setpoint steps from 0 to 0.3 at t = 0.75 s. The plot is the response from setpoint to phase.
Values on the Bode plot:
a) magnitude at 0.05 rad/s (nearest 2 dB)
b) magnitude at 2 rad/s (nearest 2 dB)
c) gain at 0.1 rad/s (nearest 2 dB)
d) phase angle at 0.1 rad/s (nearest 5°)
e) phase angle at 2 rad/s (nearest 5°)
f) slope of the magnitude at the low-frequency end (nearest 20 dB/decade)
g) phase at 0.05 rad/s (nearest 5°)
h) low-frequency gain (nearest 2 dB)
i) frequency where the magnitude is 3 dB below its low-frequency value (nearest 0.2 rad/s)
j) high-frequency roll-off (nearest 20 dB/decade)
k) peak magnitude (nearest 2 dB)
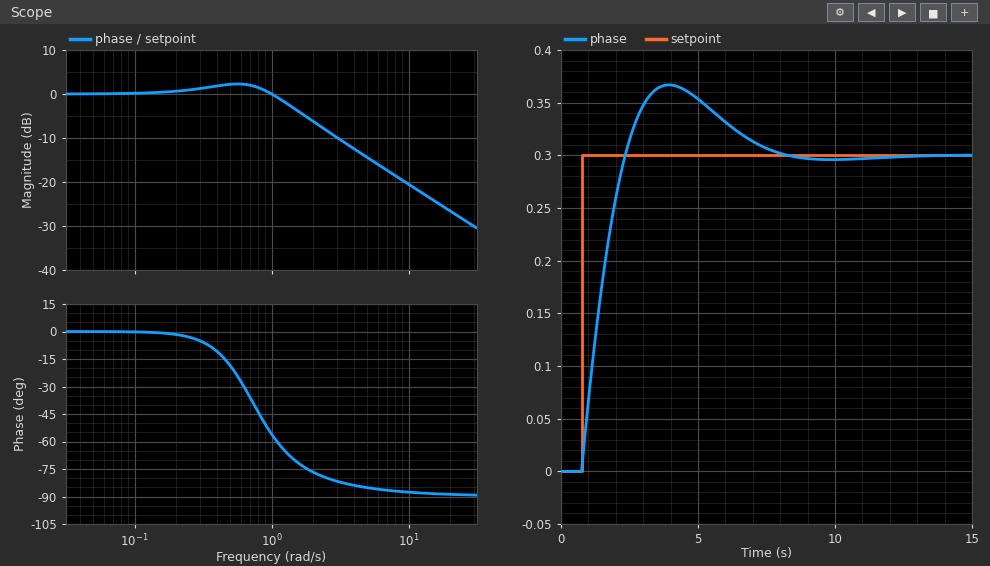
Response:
0 dB
-6 dB
0 dB
0°
-75°
0 dB/decade
0°
0 dB
1.4 rad/s
-20 dB/decade
2 dB
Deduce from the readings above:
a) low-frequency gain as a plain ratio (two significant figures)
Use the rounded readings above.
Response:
1.0
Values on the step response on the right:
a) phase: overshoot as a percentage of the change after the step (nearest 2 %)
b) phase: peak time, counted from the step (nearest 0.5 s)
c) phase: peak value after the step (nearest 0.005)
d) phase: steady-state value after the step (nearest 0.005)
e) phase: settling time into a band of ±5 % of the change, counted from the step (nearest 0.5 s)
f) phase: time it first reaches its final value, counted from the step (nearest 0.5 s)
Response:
22 %
3.0 s
0.365
0.300
6.0 s
1.5 s
